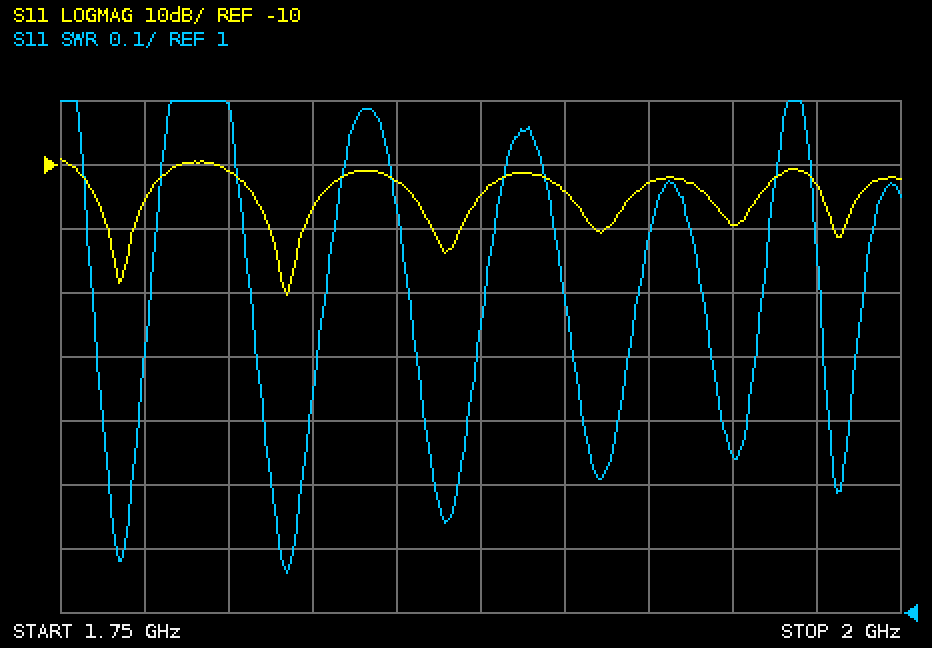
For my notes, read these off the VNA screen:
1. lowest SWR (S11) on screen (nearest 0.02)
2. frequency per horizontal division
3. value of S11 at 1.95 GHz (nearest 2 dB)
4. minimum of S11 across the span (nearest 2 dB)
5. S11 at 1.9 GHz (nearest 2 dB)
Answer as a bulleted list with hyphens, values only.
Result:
- 1.06
- 25 MHz
- -20 dB
- -30 dB
- -14 dB
